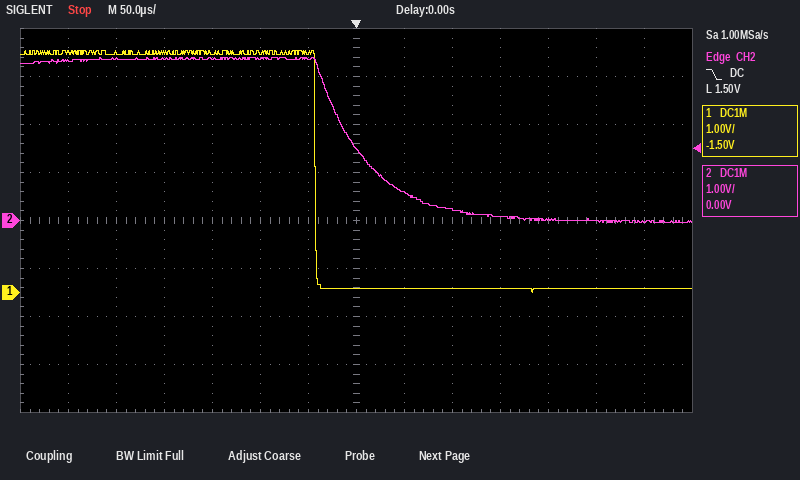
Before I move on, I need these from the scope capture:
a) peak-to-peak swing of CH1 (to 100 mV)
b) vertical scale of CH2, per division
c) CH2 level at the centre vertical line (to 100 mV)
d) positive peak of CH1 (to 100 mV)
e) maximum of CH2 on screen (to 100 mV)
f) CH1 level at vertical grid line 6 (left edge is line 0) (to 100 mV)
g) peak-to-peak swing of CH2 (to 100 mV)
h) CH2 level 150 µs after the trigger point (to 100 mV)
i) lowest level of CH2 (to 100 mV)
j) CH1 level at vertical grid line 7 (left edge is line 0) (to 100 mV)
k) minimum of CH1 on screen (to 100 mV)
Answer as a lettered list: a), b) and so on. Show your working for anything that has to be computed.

a) 5.0 V − (0.0 V) = 5.0 V
b) 1 V
c) 1.5 V
d) 5.0 V
e) 3.4 V
f) 5.0 V
g) 3.4 V − (0.0 V) = 3.4 V
h) 100 mV
i) 0.0 V
j) 100 mV
k) 0.0 V
